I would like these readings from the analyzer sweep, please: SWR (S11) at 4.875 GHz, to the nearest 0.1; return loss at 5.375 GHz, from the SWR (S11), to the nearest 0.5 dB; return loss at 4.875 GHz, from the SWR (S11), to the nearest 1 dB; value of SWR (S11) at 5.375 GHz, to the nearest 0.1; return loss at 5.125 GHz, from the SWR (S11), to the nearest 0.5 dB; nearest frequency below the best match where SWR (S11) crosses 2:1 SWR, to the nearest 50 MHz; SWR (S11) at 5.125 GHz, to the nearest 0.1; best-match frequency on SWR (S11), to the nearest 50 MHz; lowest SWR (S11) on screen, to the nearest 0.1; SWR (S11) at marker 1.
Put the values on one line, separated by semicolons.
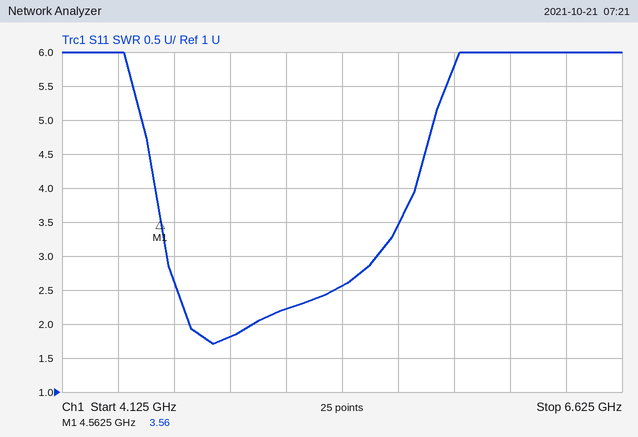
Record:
1.8; 7.0 dB; 11 dB; 2.6; 8.5 dB; 4.70 GHz; 2.2; 4.80 GHz; 1.7; 3.56
